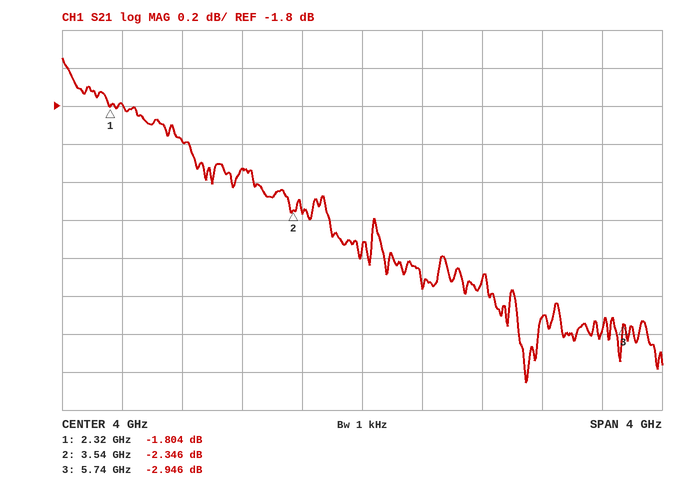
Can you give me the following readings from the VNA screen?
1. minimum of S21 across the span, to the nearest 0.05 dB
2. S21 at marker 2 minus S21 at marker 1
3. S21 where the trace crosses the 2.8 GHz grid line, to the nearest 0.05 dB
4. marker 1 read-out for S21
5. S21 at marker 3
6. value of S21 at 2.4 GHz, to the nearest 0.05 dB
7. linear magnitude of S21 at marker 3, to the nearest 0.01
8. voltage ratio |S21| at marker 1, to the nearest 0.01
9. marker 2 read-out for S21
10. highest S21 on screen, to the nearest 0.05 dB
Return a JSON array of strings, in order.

["-3.25 dB", "-0.542 dB", "-2.00 dB", "-1.804 dB", "-2.946 dB", "-1.80 dB", "0.71", "0.81", "-2.346 dB", "-1.55 dB"]
